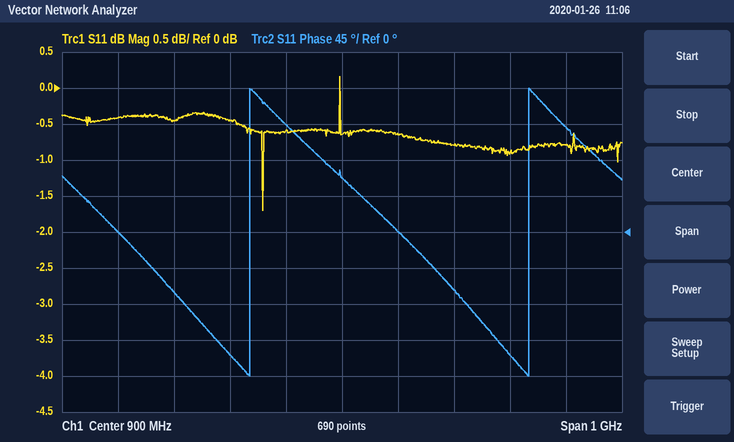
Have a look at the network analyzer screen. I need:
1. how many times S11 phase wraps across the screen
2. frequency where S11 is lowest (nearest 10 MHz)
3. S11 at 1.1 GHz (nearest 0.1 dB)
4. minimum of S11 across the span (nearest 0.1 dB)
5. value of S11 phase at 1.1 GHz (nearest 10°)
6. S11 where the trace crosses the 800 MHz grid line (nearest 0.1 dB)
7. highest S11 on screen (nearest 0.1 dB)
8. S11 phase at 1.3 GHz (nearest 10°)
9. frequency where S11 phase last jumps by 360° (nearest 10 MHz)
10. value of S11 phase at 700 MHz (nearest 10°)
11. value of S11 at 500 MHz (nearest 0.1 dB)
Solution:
2
760 MHz
-0.8 dB
-1.7 dB
-70°
-0.6 dB
0.2 dB
130°
1.23 GHz
-150°
-0.4 dB
